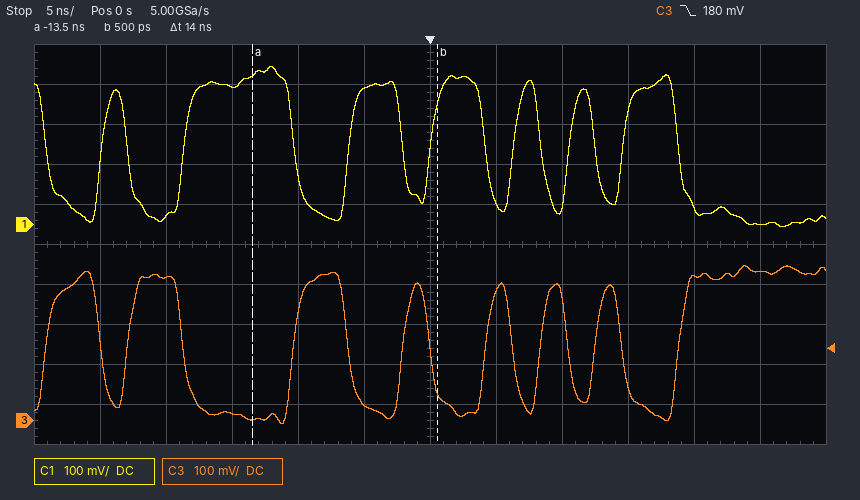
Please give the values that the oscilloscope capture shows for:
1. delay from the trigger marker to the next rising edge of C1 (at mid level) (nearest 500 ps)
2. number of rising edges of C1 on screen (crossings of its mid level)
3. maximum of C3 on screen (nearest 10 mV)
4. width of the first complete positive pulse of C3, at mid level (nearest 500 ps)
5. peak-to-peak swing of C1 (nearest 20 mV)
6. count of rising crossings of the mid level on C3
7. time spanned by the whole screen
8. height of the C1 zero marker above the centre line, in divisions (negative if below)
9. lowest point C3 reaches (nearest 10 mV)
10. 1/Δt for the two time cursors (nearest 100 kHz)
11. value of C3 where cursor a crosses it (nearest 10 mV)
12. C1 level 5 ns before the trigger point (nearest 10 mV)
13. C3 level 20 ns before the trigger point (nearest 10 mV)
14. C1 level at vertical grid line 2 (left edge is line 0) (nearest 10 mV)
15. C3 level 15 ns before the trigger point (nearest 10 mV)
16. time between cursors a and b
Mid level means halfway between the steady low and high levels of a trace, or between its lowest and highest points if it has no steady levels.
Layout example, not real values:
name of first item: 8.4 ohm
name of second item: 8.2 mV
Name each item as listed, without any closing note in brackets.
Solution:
delay from the trigger marker to the next rising edge of C1 (at mid level): 6.5 ns
number of rising edges of C1 on screen: 7
maximum of C3 on screen: 390 mV
width of the first complete positive pulse of C3, at mid level: 4.0 ns
peak-to-peak swing of C1: 400 mV
count of rising crossings of the mid level on C3: 8
time spanned by the whole screen: 60 ns
height of the C1 zero marker above the centre line, in divisions: +0.5 div
lowest point C3 reaches: -10 mV
1/Δt for the two time cursors: 71.4 MHz
value of C3 where cursor a crosses it: 0 mV
C1 level 5 ns before the trigger point: 340 mV
C3 level 20 ns before the trigger point: 360 mV
C1 level at vertical grid line 2 (left edge is line 0): 20 mV
C3 level 15 ns before the trigger point: 20 mV
time between cursors a and b: 14 ns
